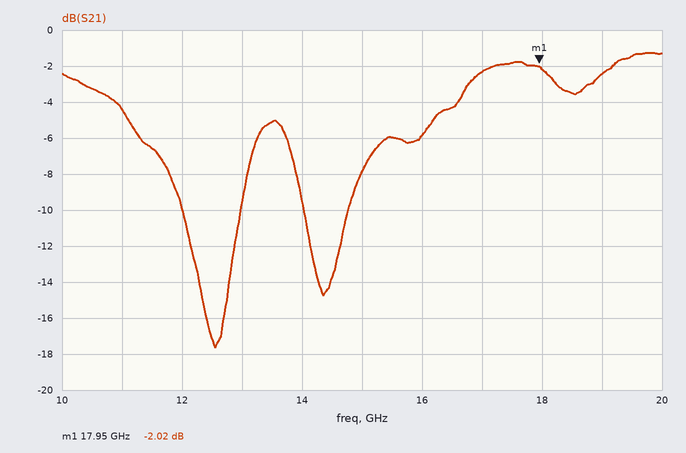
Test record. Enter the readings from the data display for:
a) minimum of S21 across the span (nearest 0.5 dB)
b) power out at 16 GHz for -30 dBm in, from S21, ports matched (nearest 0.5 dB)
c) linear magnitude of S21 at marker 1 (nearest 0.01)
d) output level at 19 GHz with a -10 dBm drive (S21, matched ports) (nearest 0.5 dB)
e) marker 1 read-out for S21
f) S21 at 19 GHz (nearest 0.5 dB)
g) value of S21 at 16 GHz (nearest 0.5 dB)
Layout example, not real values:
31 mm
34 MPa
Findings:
-17.5 dB
-36.0 dBm
0.79
-12.5 dBm
-2.02 dB
-2.5 dB
-6.0 dB
